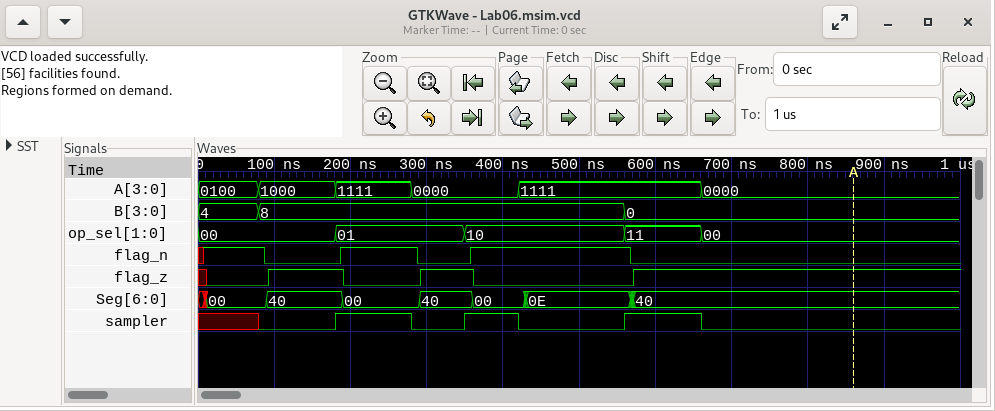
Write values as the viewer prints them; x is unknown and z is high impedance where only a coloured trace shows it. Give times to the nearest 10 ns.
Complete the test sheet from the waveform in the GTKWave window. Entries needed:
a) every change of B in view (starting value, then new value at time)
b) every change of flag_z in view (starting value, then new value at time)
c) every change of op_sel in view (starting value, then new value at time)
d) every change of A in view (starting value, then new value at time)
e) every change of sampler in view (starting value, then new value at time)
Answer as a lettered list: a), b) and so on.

a) 4, 8 at 80 ns, 0 at 560 ns
b) x, 0 at 10 ns, 1 at 90 ns, 0 at 190 ns, 1 at 290 ns, 0 at 360 ns, 1 at 570 ns
c) 00, 01 at 180 ns, 10 at 350 ns, 11 at 560 ns, 00 at 660 ns
d) 0100, 1000 at 80 ns, 1111 at 180 ns, 0000 at 280 ns, 1111 at 420 ns, 0000 at 660 ns
e) x, 0 at 80 ns, 1 at 180 ns, 0 at 280 ns, 1 at 350 ns, 0 at 420 ns, 1 at 560 ns, 0 at 660 ns
